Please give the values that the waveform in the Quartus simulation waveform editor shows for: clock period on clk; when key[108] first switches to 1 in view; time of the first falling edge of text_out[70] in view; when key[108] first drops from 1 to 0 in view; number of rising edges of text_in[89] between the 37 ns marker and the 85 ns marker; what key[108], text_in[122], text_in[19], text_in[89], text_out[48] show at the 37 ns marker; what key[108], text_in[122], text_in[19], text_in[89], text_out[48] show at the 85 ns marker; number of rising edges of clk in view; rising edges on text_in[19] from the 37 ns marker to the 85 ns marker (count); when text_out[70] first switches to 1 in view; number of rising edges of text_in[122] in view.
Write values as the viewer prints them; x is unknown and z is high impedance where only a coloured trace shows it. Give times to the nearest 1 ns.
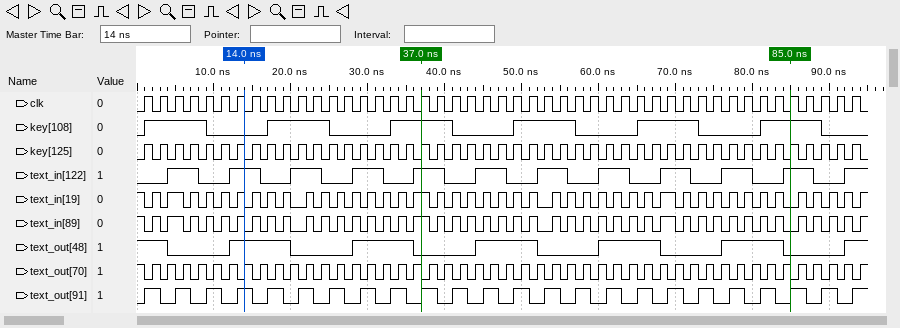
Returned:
2 ns
1 ns
1 ns
9 ns
22
key[108]=1, text_in[122]=1, text_in[19]=1, text_in[89]=1, text_out[48]=0
key[108]=1, text_in[122]=1, text_in[19]=0, text_in[89]=0, text_out[48]=0
47
22
2 ns
12
